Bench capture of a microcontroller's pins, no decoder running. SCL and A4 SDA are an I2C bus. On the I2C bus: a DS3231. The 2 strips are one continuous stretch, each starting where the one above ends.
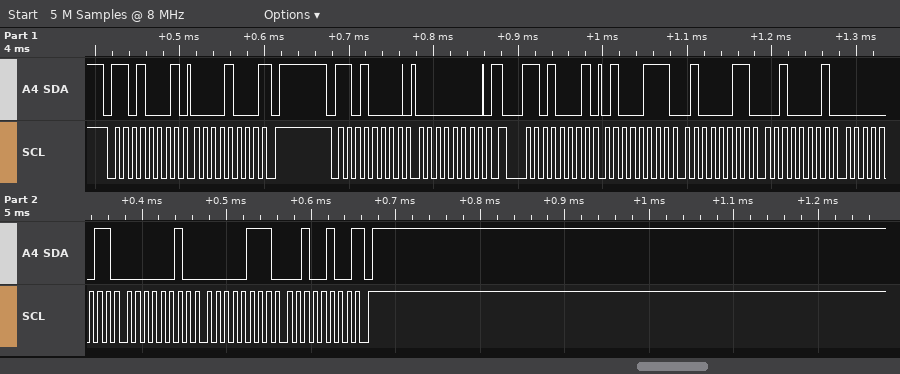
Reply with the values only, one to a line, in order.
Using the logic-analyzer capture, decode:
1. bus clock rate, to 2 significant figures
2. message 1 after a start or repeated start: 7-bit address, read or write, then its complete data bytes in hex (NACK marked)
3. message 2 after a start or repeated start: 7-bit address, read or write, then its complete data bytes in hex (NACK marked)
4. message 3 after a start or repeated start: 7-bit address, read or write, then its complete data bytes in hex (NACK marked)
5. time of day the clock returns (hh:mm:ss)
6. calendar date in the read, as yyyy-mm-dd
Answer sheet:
100 kHz
0x68 read: 08 NACK
0x68 write: 00
0x68 read: 47 43 21 03 02 07 24 NACK
21:43:47
2024-07-02
